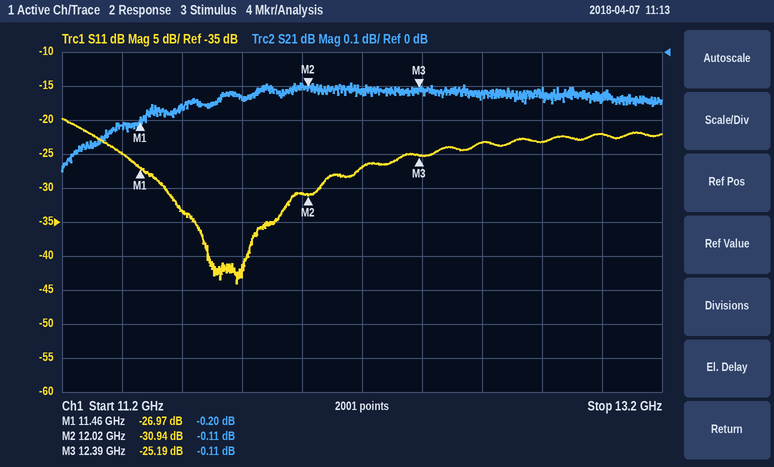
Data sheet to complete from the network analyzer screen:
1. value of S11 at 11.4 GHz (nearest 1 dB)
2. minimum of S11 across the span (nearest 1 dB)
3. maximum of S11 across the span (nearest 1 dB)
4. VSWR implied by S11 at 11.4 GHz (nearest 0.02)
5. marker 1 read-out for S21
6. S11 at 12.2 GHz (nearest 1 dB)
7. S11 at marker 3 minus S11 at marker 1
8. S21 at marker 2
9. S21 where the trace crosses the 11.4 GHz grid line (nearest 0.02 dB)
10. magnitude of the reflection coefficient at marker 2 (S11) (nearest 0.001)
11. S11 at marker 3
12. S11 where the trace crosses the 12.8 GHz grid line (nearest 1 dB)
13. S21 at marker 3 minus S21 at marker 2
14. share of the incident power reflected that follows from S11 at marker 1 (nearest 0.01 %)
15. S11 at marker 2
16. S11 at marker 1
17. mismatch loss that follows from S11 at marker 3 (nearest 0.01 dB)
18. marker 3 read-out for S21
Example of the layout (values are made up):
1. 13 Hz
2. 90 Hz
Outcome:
1. -25 dB
2. -44 dB
3. -20 dB
4. 1.12
5. -0.20 dB
6. -27 dB
7. 1.78 dB
8. -0.11 dB
9. -0.22 dB
10. 0.028
11. -25.19 dB
12. -23 dB
13. 0.00 dB
14. 0.20 %
15. -30.94 dB
16. -26.97 dB
17. 0.01 dB
18. -0.11 dB
